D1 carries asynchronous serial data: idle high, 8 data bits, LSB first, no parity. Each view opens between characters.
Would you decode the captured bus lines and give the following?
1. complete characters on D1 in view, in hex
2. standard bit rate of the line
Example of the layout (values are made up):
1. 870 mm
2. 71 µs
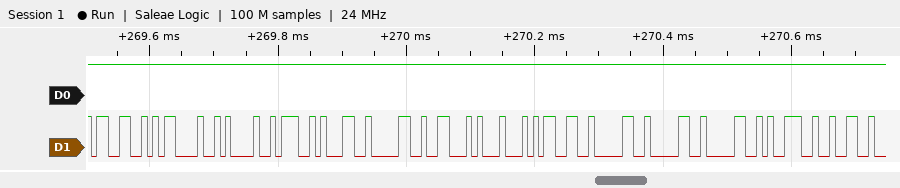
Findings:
1. 33, 0D, 0A, 3A, 31, 30, 46, 44, 33, 30, 30, 30, 39, 32
2. 115200 baud
